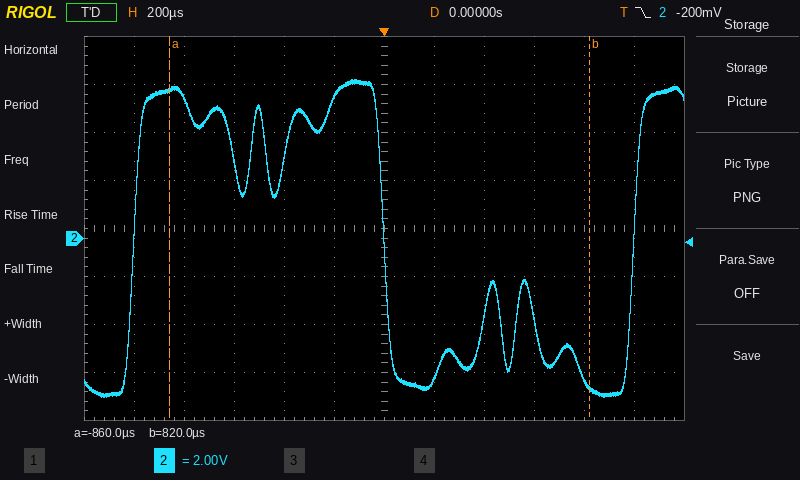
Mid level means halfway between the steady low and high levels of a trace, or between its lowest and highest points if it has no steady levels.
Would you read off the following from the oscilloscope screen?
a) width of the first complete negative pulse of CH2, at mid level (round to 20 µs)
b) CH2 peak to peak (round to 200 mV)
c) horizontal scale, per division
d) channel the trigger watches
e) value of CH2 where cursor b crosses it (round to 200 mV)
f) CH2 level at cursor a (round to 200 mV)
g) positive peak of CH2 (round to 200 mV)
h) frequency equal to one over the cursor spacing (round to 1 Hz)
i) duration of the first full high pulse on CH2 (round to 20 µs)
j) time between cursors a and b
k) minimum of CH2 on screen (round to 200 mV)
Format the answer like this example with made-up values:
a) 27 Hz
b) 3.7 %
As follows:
a) 1.00 ms
b) 13.2 V
c) 200 µs
d) CH2
e) -6.2 V
f) 6.2 V
g) 6.6 V
h) 595 Hz
i) 1.00 ms
j) 1.68 ms
k) -6.6 V
